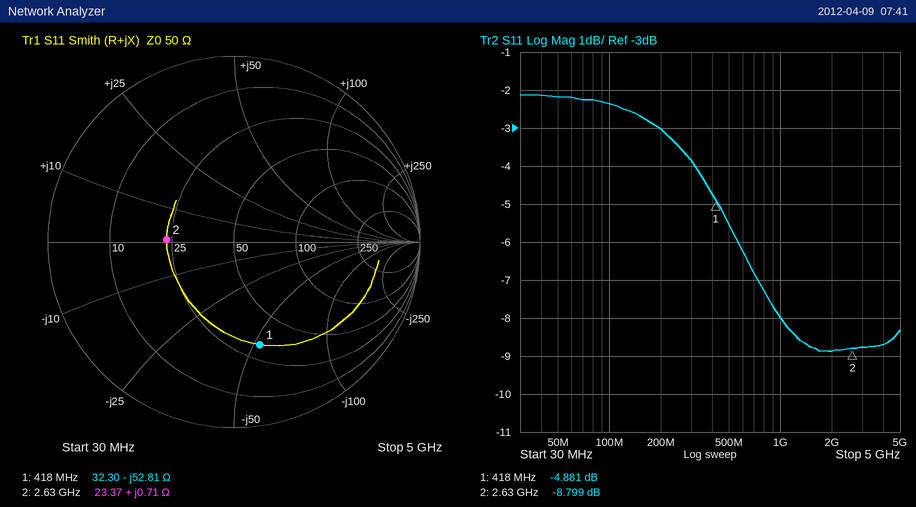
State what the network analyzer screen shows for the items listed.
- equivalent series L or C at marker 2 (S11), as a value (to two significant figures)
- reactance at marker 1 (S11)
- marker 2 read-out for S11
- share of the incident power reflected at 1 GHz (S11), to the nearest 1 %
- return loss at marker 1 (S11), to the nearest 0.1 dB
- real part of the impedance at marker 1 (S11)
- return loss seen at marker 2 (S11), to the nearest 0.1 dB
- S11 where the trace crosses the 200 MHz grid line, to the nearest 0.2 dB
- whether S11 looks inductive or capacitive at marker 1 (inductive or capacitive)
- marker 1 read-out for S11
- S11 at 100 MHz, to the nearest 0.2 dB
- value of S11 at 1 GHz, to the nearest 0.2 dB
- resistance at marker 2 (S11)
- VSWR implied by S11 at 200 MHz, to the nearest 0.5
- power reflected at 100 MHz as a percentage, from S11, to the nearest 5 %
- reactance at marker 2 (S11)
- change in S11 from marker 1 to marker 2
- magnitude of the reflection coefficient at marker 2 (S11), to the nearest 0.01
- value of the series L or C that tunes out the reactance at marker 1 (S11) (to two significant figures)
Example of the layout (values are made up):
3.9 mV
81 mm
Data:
43 pH
-52.81 Ω
-8.799 dB
16 %
4.9 dB
32.30 Ω
8.8 dB
-3.0 dB
capacitive
-4.881 dB
-2.4 dB
-8.0 dB
23.37 Ω
6.0
60 %
+0.71 Ω
-3.918 dB
0.36
20 nH
